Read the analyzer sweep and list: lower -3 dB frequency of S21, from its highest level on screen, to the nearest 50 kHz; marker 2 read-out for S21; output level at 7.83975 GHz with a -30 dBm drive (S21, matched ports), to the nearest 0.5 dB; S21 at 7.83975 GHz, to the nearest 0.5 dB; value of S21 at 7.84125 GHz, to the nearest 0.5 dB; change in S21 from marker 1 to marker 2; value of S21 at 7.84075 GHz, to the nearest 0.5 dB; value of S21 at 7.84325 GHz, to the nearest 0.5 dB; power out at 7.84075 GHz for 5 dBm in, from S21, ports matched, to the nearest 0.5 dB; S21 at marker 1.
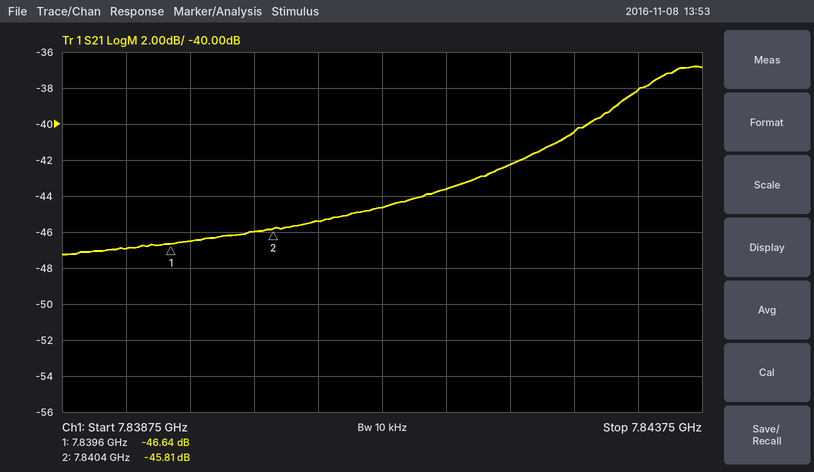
7.84290 GHz
-45.81 dB
-76.5 dBm
-46.5 dB
-44.5 dB
0.83 dB
-45.5 dB
-38.0 dB
-40.5 dBm
-46.64 dB
